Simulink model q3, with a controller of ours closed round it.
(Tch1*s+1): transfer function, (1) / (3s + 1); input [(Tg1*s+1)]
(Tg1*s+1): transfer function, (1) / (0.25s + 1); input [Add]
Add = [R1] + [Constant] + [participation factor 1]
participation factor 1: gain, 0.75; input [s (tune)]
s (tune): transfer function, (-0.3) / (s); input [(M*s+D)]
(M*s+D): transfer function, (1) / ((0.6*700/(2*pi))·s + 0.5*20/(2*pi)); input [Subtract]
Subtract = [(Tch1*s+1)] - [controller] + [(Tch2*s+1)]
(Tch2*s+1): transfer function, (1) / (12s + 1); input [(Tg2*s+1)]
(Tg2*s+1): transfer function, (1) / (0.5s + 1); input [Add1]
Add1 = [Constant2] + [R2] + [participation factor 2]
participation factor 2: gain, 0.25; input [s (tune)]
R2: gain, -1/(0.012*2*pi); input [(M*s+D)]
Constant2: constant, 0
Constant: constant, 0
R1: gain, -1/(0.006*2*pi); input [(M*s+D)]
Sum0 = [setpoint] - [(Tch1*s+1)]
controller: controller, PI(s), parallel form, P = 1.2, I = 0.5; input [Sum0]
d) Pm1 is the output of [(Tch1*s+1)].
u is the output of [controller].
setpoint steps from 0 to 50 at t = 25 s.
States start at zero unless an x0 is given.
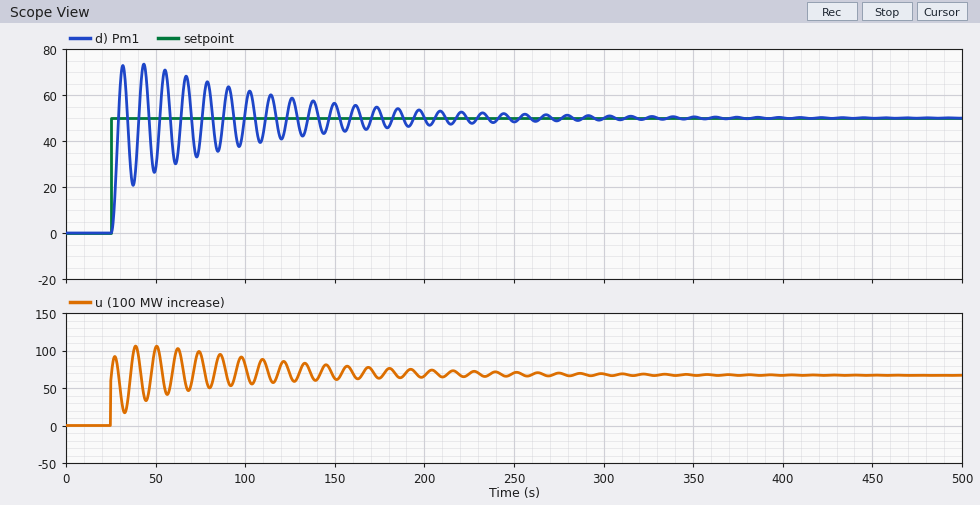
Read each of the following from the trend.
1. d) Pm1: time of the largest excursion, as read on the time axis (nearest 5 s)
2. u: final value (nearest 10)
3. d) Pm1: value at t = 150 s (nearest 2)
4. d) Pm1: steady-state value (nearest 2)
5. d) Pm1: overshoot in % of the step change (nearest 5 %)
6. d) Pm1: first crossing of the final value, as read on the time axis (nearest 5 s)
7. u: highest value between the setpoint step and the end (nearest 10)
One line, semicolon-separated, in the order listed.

45 s; 70; 56; 50; 45 %; 30 s; 110
